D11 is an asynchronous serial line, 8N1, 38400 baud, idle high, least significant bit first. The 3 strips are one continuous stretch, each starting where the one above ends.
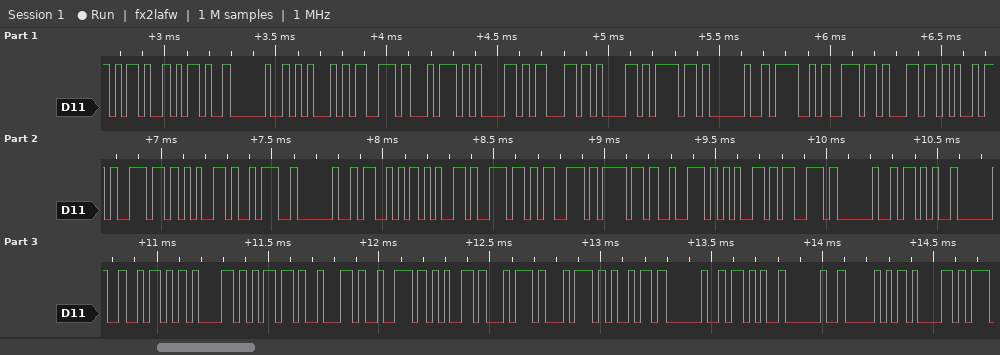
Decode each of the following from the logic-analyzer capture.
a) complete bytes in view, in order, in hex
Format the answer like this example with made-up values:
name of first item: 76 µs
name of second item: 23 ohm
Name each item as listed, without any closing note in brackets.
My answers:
complete bytes in view, in order, in hex: 2D 2D 20 45 73 74 61 63 61 6F 20 4F 6E 6C 69 6E 65 3A 20 53 65 6E 73 6F 72 65 73 20 2B 20 5A 61 6D 62 72 65 74 74 69 20 2B 20 50 61
